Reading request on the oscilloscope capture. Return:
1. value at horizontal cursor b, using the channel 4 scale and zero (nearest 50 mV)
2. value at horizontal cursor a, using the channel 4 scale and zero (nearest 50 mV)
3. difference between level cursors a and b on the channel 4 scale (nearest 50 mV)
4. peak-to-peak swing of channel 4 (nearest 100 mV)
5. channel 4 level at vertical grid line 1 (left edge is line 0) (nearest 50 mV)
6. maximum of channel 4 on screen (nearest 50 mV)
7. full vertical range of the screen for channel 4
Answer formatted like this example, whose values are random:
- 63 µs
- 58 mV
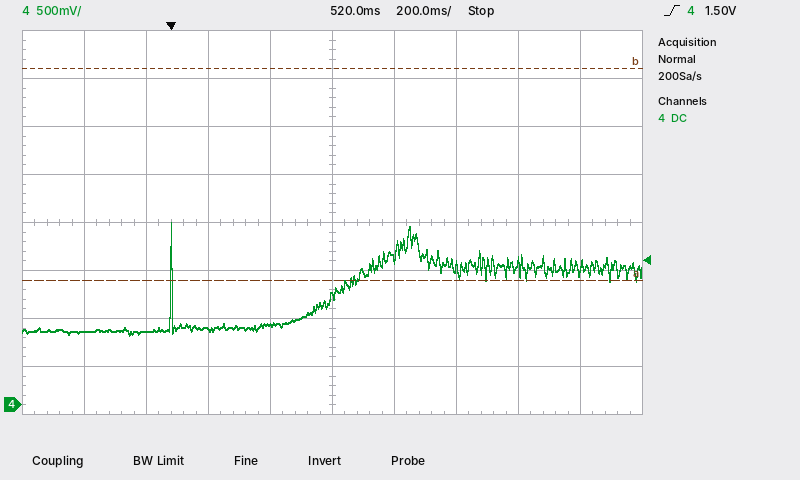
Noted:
- 3.50 V
- 1.30 V
- 2.20 V
- 1.20 V
- 750 mV
- 1.90 V
- 4 V
